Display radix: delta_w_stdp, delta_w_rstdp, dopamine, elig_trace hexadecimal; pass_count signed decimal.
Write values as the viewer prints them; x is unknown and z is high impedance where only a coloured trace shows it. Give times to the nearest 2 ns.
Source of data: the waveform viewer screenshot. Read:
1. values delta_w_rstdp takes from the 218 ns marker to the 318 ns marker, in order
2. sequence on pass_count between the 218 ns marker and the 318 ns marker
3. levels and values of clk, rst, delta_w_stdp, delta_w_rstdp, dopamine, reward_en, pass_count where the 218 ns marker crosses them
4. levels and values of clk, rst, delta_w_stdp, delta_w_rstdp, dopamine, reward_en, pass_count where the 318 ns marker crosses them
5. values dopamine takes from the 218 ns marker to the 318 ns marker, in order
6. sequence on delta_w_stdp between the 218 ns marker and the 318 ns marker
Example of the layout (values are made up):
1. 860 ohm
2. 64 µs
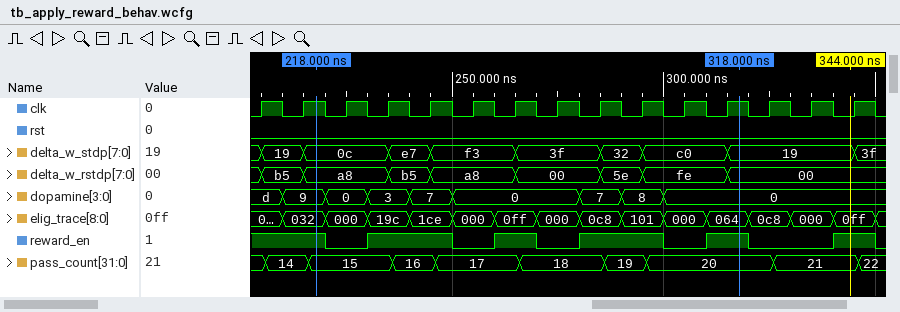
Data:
1. a8, b5, a8, 00, 5e, fe, 00
2. 15, 16, 17, 18, 19, 20
3. clk=1, rst=0, delta_w_stdp=0c, delta_w_rstdp=a8, dopamine=9, reward_en=1, pass_count=15
4. clk=1, rst=0, delta_w_stdp=19, delta_w_rstdp=00, dopamine=0, reward_en=1, pass_count=20
5. 9, 0, 3, 7, 0, 7, 8, 0
6. 0c, e7, f3, 3f, 32, c0, 19
